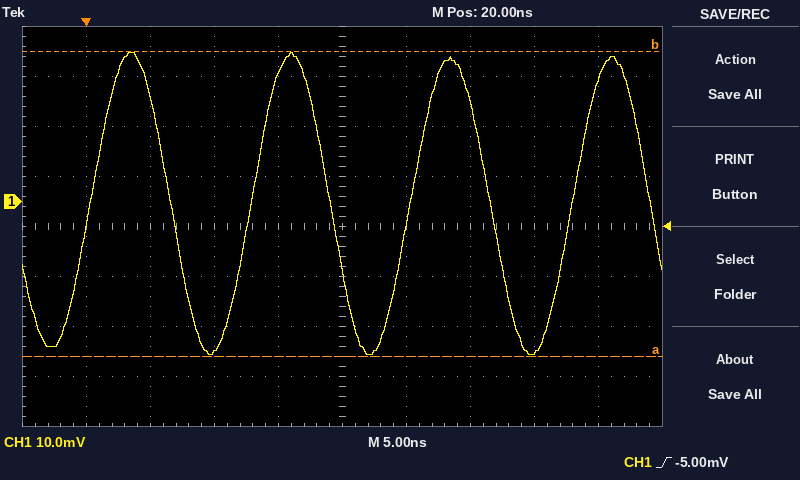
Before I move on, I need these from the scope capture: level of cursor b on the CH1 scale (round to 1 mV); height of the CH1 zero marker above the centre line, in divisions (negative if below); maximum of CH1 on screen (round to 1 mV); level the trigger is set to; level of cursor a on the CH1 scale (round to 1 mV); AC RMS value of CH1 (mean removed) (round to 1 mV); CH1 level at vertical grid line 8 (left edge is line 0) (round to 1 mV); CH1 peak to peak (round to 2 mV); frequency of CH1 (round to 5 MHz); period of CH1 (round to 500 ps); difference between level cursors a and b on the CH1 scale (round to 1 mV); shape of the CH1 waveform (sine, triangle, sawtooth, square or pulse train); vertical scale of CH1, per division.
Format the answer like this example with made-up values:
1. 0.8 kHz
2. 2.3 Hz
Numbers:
1. 30 mV
2. +0.5 div
3. 30 mV
4. -5.00 mV
5. -31 mV
6. 21 mV
7. -30 mV
8. 60 mV
9. 80 MHz
10. 12.5 ns
11. 61 mV
12. sine
13. 10 mV
